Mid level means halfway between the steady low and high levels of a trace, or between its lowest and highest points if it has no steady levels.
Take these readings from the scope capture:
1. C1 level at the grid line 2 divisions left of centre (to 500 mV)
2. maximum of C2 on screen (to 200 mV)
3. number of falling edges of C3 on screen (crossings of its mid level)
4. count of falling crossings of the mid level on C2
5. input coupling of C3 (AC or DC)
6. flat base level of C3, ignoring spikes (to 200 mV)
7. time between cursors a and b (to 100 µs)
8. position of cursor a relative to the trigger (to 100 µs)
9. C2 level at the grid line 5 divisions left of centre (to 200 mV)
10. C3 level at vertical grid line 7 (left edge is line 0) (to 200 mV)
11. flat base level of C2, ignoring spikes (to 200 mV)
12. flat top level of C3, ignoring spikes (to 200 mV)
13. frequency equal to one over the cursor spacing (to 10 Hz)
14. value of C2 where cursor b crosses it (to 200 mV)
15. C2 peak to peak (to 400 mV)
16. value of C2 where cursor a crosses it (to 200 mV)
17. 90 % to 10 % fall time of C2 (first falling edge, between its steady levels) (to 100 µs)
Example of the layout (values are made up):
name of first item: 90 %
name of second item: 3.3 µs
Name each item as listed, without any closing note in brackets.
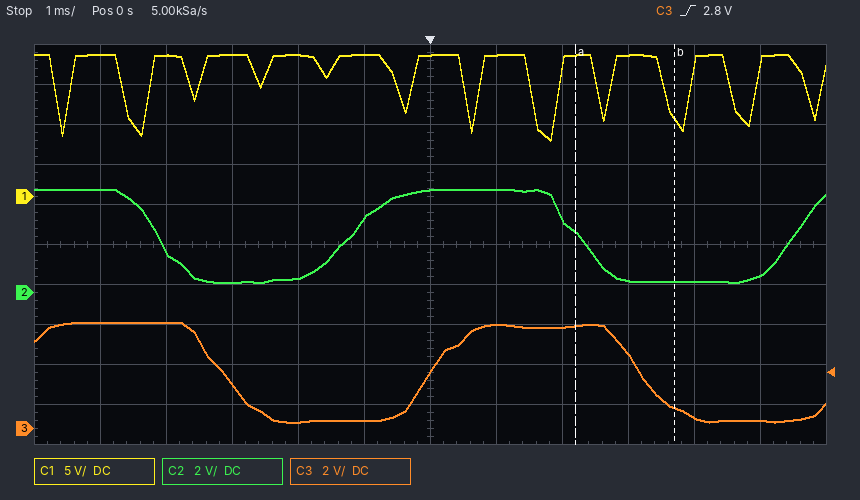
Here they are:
C1 level at the grid line 2 divisions left of centre: 17.5 V
maximum of C2 on screen: 5.2 V
number of falling edges of C3 on screen: 2
count of falling crossings of the mid level on C2: 2
input coupling of C3: DC
flat base level of C3, ignoring spikes: 400 mV
time between cursors a and b: 1.5 ms
position of cursor a relative to the trigger: +2.2 ms
C2 level at the grid line 5 divisions left of centre: 5.2 V
C3 level at vertical grid line 7 (left edge is line 0): 5.2 V
flat base level of C2, ignoring spikes: 600 mV
flat top level of C3, ignoring spikes: 5.2 V
frequency equal to one over the cursor spacing: 670 Hz
value of C2 where cursor b crosses it: 600 mV
C2 peak to peak: 4.8 V
value of C2 where cursor a crosses it: 3.0 V
90 % to 10 % fall time of C2 (first falling edge, between its steady levels): 900 µs
